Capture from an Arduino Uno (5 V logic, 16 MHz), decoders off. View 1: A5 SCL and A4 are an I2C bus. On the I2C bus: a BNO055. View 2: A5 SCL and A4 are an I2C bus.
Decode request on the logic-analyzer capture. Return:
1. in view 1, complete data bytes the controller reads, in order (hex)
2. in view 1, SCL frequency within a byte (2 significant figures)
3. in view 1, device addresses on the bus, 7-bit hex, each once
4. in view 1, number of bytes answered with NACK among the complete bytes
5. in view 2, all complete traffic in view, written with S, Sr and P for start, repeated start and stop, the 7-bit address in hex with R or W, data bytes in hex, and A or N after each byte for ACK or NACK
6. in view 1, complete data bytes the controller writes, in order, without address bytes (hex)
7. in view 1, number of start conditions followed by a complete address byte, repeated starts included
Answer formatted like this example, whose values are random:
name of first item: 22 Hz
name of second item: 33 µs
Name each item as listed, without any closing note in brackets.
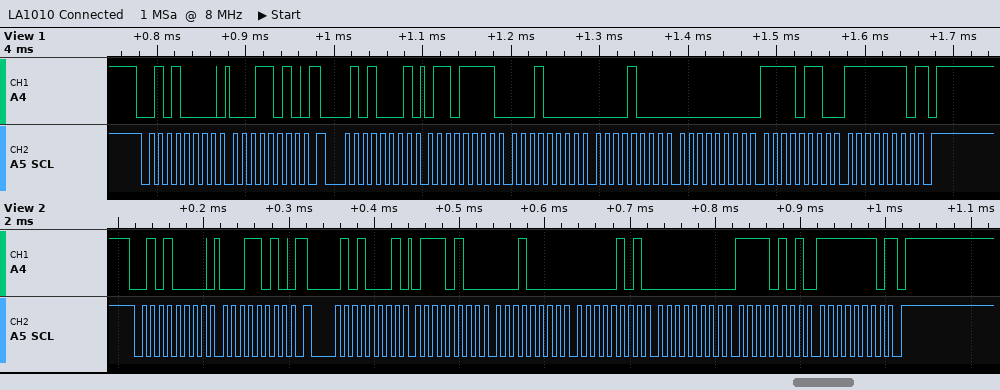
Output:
in view 1, complete data bytes the controller reads, in order: 6F 10 08 00 F6 FE
in view 1, SCL frequency within a byte: 100 kHz
in view 1, device addresses on the bus, 7-bit hex, each once: 0x28
in view 1, number of bytes answered with NACK among the complete bytes: 1
in view 2, all complete traffic in view, written with S, Sr and P for start, repeated start and stop, the 7-bit address in hex with R or W, data bytes in hex, and A or N after each byte for ACK or NACK: S 28W A 1A A Sr 28R A 74 A 10 A 05 A 00 A F5 A FE N P
in view 1, complete data bytes the controller writes, in order, without address bytes: 1A
in view 1, number of start conditions followed by a complete address byte, repeated starts included: 2
